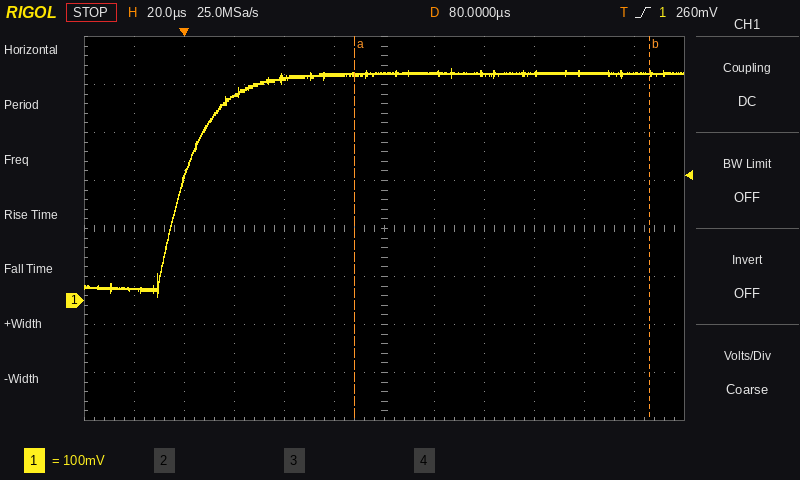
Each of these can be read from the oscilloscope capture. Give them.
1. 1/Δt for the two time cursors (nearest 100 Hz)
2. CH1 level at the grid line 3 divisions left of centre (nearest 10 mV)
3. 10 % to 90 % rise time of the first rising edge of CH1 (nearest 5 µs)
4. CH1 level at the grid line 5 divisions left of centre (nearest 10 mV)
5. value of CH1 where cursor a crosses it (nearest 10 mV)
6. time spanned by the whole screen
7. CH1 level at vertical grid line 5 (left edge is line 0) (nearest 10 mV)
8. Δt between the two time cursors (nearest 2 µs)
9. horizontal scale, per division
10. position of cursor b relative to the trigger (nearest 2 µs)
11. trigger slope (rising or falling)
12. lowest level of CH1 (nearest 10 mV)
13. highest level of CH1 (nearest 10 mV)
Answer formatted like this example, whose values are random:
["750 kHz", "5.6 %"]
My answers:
["8.5 kHz", "430 mV", "30 µs", "20 mV", "470 mV", "240 µs", "470 mV", "118 µs", "20 µs", "+186 µs", "rising", "10 mV", "480 mV"]
